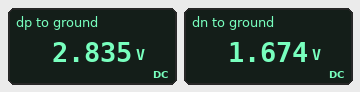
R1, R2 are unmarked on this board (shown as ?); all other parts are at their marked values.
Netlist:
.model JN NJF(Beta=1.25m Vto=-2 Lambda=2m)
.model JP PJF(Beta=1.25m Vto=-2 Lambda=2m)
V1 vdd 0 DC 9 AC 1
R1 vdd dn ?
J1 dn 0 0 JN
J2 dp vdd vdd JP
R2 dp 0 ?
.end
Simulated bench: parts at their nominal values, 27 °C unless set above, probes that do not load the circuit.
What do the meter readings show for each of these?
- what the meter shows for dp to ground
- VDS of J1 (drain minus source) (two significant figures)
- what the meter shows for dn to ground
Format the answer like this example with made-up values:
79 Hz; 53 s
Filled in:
2.835 V; 1.7 V; 1.674 V
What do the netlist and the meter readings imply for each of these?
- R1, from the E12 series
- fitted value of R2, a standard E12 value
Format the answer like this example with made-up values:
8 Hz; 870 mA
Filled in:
1.5 kΩ; 560 Ω
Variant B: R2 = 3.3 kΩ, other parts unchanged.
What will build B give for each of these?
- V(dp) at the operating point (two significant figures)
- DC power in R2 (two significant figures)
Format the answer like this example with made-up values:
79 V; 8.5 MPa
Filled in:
8.4 V; 21 mW
